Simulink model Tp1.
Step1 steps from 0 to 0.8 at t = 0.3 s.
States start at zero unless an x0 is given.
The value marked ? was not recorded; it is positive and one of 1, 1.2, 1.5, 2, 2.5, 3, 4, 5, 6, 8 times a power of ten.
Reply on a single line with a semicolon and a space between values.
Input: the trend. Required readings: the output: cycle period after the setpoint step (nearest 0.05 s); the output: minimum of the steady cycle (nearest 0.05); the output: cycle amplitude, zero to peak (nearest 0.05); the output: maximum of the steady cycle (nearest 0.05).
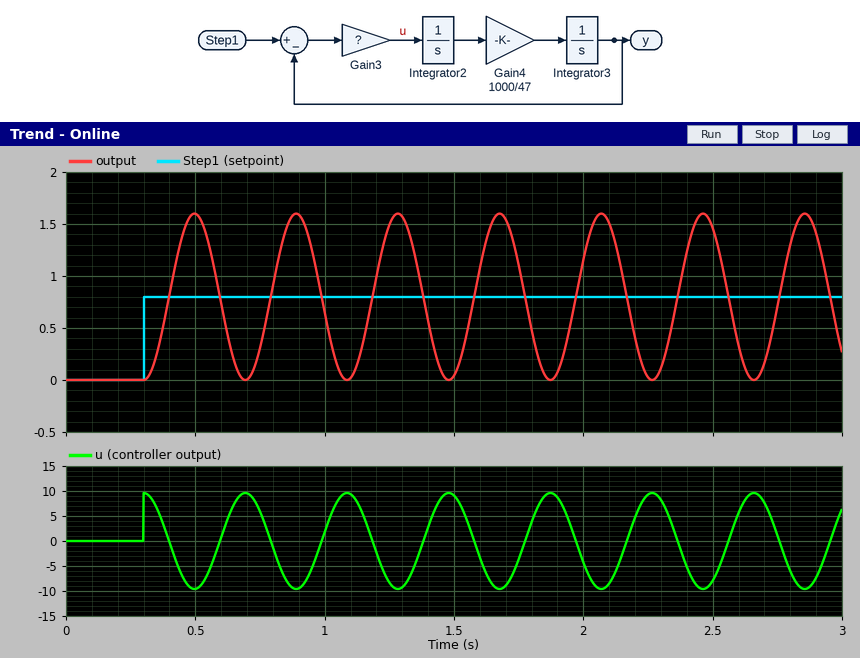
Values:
0.40 s; 0.00; 0.80; 1.60
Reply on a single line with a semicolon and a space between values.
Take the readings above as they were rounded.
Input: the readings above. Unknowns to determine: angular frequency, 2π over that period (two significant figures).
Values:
16 rad/s
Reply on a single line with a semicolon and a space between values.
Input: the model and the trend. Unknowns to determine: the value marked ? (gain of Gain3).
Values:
12
